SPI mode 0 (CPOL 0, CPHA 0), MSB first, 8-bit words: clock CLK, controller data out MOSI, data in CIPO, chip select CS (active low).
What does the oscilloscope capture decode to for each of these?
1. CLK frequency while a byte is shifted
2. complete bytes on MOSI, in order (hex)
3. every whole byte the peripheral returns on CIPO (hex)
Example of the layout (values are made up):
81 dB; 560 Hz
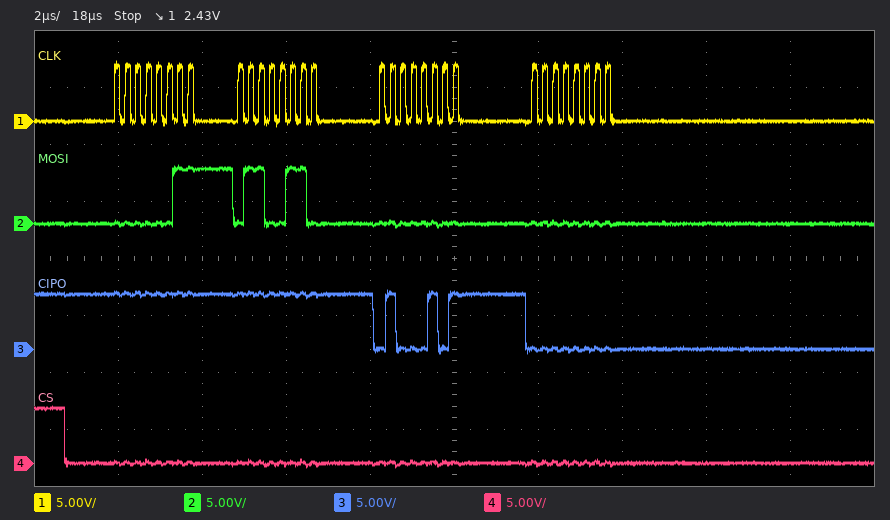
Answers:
4 MHz; 03 66 00 00; FF FF 45 00
